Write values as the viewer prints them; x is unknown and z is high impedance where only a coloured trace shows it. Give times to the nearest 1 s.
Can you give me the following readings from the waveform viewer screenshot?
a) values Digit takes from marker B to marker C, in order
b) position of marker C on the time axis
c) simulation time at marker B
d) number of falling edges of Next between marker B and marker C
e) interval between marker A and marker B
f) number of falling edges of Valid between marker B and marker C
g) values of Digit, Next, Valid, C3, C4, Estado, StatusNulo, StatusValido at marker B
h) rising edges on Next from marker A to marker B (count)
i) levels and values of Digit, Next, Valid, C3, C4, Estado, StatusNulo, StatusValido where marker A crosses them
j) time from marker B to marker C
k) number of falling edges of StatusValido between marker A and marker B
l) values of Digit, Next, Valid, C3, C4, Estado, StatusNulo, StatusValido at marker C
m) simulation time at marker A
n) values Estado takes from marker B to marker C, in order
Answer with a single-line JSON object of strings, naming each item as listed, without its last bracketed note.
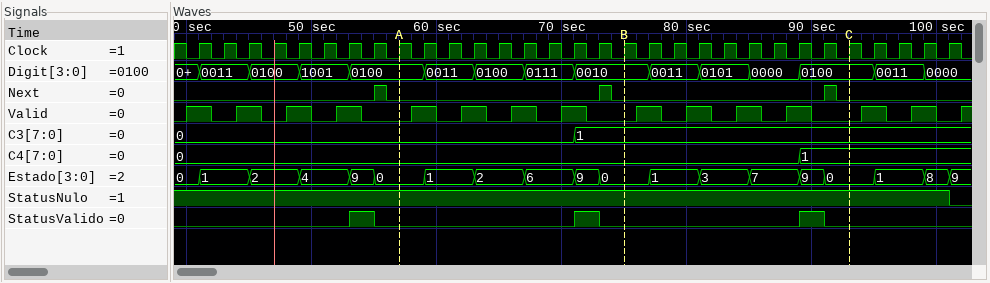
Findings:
{"values Digit takes from marker B to marker C, in order": "0010, 0011, 0101, 0000, 0100", "position of marker C on the time axis": "93 s", "simulation time at marker B": "75 s", "number of falling edges of Next between marker B and marker C": "1", "interval between marker A and marker B": "18 s", "number of falling edges of Valid between marker B and marker C": "4", "values of Digit, Next, Valid, C3, C4, Estado, StatusNulo, StatusValido at marker B": "Digit=0010, Next=0, Valid=0, C3=1, C4=0, Estado=0, StatusNulo=1, StatusValido=0", "rising edges on Next from marker A to marker B": "1", "levels and values of Digit, Next, Valid, C3, C4, Estado, StatusNulo, StatusValido where marker A crosses them": "Digit=0100, Next=0, Valid=0, C3=0, C4=0, Estado=0, StatusNulo=1, StatusValido=0", "time from marker B to marker C": "18 s", "number of falling edges of StatusValido between marker A and marker B": "1", "values of Digit, Next, Valid, C3, C4, Estado, StatusNulo, StatusValido at marker C": "Digit=0100, Next=0, Valid=0, C3=1, C4=1, Estado=0, StatusNulo=1, StatusValido=0", "simulation time at marker A": "57 s", "values Estado takes from marker B to marker C, in order": "0, 1, 3, 7, 9, 0"}
